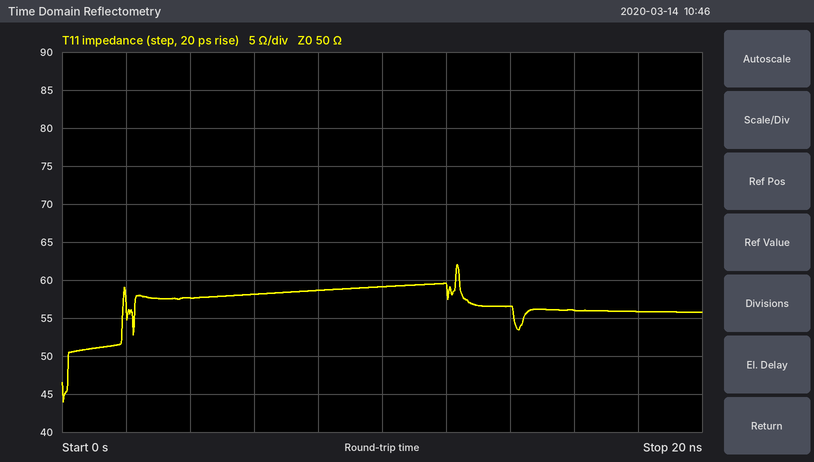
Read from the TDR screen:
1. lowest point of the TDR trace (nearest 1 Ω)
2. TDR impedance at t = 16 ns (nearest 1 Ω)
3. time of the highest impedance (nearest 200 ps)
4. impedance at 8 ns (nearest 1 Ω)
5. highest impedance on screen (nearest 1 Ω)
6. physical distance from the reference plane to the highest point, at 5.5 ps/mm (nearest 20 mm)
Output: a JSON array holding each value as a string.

["44 Ω", "56 Ω", "12.4 ns", "59 Ω", "62 Ω", "1.12 m"]
